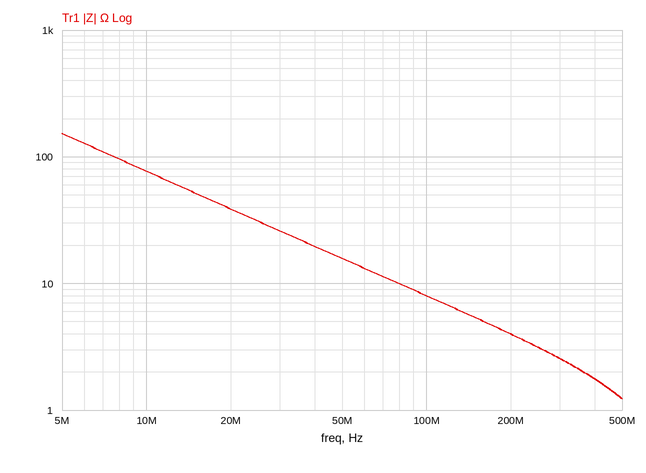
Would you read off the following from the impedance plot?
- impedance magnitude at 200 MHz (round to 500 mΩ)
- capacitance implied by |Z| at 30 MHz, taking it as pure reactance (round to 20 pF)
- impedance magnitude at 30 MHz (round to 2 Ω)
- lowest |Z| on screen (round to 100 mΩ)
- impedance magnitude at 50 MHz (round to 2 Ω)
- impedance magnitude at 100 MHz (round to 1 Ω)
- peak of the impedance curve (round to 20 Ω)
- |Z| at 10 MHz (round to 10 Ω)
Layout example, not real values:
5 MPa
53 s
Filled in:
4.0 Ω
200 pF
26 Ω
1.2 Ω
16 Ω
8 Ω
160 Ω
80 Ω
